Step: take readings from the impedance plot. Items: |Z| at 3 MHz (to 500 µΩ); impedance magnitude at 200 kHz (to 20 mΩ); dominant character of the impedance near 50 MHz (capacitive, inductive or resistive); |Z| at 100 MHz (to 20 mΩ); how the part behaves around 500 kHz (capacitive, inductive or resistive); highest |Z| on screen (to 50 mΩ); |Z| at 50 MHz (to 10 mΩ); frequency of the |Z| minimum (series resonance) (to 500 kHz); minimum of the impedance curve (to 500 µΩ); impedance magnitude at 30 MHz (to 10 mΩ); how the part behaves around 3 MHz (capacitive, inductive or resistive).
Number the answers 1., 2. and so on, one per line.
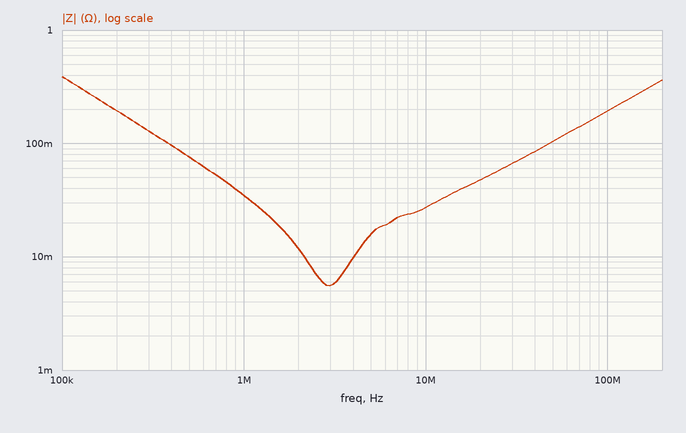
1. 5.5 mΩ
2. 200 mΩ
3. inductive
4. 200 mΩ
5. capacitive
6. 400 mΩ
7. 100 mΩ
8. 3.0 MHz
9. 5.5 mΩ
10. 70 mΩ
11. resistive
